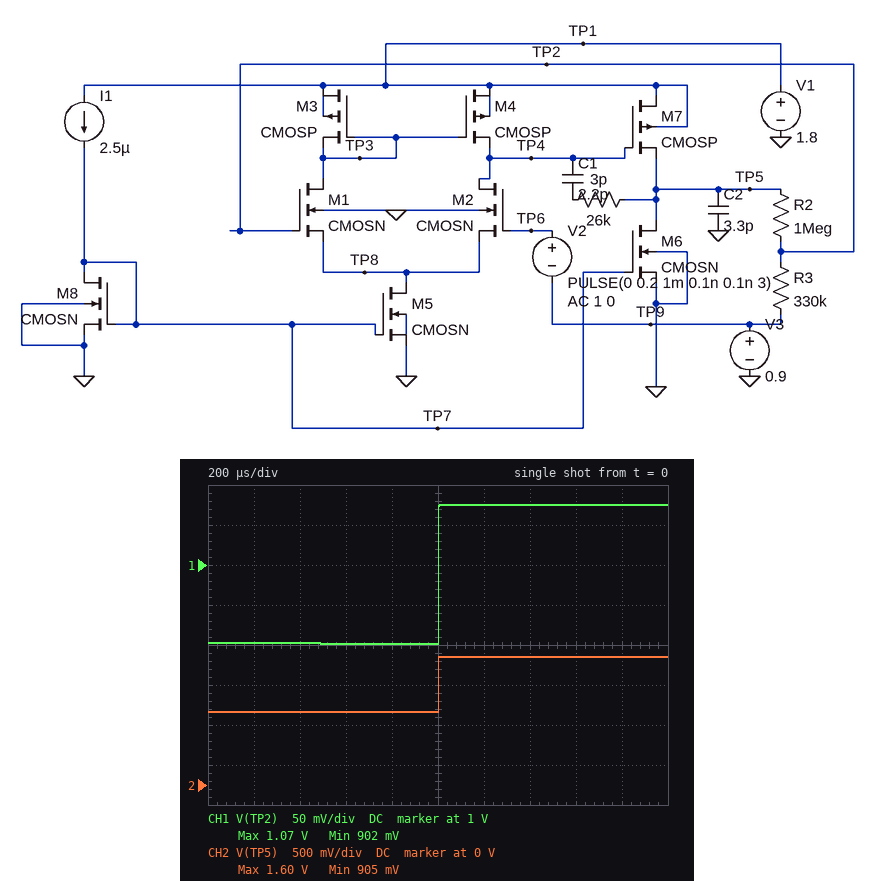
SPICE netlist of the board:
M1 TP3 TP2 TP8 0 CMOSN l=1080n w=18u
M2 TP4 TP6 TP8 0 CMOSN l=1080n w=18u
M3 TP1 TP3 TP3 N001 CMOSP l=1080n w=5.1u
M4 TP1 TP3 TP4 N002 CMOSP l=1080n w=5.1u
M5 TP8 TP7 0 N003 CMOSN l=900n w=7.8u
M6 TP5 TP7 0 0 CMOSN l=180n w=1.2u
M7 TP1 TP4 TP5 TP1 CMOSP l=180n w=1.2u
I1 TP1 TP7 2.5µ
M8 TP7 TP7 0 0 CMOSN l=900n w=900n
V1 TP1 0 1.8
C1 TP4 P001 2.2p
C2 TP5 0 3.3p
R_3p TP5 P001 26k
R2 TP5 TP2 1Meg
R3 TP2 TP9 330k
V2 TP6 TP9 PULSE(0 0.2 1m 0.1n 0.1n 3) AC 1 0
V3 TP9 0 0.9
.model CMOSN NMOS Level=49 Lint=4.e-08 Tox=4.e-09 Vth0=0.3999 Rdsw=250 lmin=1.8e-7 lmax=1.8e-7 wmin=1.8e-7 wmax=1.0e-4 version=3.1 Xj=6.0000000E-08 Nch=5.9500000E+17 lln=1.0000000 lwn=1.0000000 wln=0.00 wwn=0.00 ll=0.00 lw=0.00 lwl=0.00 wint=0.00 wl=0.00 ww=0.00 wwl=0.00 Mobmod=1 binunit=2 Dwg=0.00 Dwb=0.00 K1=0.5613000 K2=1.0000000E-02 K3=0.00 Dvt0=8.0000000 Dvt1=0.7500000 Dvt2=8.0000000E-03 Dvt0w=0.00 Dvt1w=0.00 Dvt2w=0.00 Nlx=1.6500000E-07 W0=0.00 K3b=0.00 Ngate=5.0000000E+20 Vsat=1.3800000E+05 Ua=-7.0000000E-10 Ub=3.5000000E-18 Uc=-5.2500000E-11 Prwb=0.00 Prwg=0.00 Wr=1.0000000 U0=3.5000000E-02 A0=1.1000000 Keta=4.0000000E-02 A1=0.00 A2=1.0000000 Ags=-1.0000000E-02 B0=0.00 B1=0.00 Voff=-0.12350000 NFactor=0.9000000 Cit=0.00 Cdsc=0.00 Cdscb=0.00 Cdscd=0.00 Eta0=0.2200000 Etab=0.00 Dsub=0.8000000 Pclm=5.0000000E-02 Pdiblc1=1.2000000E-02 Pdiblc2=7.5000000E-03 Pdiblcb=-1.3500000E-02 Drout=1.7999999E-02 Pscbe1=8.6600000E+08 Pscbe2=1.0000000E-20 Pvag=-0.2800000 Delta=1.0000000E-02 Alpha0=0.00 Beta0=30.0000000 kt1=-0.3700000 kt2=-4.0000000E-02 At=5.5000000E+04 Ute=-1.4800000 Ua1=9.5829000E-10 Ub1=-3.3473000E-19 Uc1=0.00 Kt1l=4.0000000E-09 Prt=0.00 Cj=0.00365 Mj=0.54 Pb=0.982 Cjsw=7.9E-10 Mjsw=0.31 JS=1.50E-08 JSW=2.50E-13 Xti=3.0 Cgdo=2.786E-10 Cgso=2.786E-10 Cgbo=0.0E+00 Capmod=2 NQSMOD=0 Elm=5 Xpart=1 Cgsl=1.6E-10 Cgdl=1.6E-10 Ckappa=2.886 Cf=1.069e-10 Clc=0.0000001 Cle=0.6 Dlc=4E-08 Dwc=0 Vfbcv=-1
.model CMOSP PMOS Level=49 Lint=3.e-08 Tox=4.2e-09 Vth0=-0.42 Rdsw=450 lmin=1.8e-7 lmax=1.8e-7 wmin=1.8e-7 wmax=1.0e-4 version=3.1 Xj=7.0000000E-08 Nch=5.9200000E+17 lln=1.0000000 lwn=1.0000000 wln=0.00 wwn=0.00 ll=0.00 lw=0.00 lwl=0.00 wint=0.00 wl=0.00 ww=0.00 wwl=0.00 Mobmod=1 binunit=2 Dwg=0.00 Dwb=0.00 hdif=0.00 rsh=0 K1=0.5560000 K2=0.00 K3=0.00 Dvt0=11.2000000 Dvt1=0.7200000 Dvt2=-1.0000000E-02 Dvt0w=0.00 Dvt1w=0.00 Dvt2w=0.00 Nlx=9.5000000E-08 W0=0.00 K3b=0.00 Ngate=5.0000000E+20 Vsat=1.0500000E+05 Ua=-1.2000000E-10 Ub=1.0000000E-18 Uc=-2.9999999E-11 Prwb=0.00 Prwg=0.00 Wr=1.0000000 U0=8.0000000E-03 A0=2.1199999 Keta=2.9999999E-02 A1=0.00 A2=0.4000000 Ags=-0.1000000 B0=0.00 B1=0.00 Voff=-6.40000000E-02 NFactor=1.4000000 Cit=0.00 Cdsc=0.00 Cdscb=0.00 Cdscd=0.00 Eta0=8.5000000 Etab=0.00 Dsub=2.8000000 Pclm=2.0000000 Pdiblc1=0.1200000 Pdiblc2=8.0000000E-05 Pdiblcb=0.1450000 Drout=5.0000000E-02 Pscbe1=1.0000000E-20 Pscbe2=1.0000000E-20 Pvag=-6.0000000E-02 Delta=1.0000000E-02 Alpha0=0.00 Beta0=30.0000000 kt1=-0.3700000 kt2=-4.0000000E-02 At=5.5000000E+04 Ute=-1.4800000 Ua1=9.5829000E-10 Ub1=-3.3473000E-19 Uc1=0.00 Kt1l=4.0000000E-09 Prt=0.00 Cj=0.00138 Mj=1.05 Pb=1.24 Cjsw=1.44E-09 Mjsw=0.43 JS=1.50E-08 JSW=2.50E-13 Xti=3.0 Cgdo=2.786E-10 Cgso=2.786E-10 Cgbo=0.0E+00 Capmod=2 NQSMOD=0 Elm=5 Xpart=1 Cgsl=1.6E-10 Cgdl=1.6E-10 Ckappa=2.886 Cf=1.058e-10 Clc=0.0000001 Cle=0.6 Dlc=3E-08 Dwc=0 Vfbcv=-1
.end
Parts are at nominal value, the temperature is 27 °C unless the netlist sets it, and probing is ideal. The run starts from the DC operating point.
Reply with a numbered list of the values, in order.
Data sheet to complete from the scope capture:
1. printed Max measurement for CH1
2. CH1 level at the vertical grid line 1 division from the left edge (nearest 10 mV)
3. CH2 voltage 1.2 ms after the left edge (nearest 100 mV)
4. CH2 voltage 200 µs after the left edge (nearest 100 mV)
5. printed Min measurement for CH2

1. 1.07 V
2. 900 mV
3. 1.6 V
4. 900 mV
5. 905 mV
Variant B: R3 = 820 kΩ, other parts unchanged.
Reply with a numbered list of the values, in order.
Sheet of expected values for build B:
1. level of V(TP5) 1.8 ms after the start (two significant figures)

1. 1.3 V
